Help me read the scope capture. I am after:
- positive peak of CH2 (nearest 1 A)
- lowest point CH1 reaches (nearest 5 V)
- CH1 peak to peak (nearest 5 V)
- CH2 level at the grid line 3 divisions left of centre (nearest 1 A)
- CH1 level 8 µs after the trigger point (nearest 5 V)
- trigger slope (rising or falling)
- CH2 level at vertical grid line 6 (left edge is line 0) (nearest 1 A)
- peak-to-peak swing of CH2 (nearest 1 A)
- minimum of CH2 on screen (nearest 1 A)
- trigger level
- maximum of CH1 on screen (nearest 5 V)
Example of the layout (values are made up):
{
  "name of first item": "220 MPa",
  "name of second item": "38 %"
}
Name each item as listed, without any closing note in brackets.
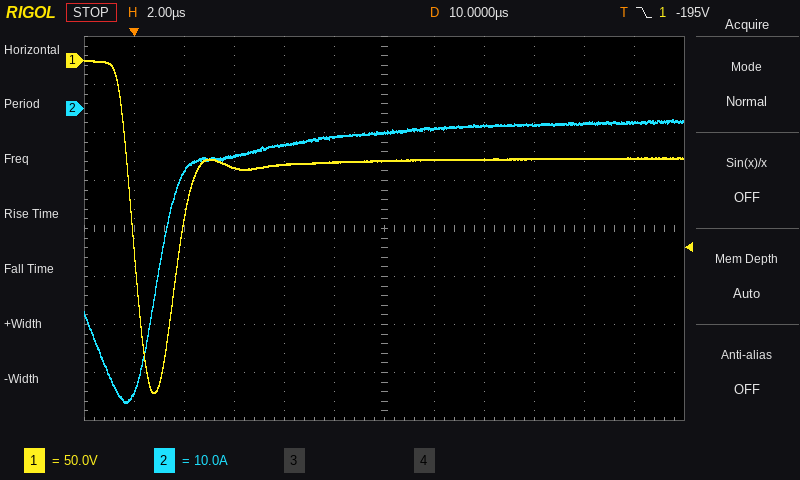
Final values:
{
  "positive peak of CH2": "-2 A",
  "lowest point CH1 reaches": "-345 V",
  "CH1 peak to peak": "345 V",
  "CH2 level at the grid line 3 divisions left of centre": "-10 A",
  "CH1 level 8 µs after the trigger point": "-105 V",
  "trigger slope": "falling",
  "CH2 level at vertical grid line 6 (left edge is line 0)": "-5 A",
  "peak-to-peak swing of CH2": "59 A",
  "minimum of CH2 on screen": "-61 A",
  "trigger level": "-195 V",
  "maximum of CH1 on screen": "0 V"
}
